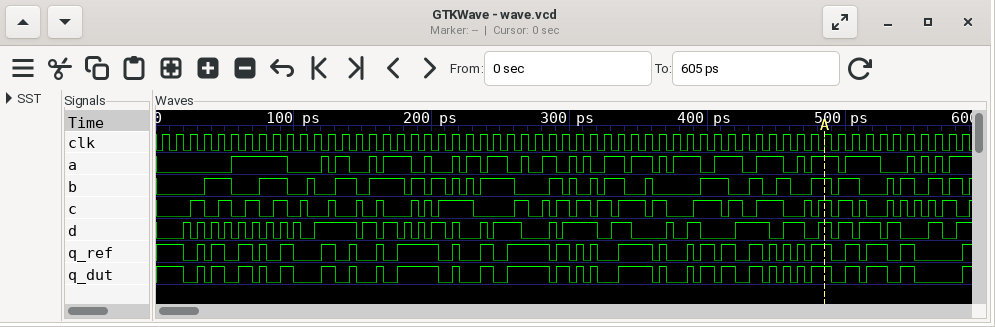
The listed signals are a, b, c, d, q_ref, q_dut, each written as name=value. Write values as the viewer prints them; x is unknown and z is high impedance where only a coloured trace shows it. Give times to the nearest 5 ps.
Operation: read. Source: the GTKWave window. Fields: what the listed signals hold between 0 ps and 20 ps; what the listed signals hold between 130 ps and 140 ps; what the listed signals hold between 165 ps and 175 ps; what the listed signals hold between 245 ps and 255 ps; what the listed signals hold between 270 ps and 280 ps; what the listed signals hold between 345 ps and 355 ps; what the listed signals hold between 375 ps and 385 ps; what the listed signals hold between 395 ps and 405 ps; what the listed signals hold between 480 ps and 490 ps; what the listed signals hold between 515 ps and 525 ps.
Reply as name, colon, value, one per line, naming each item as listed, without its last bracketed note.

what the listed signals hold between 0 ps and 20 ps: a=0, b=0, c=0, d=0, q_ref=1, q_dut=1
what the listed signals hold between 130 ps and 140 ps: a=1, b=1, c=0, d=1, q_ref=0, q_dut=0
what the listed signals hold between 165 ps and 175 ps: a=1, b=1, c=0, d=1, q_ref=0, q_dut=0
what the listed signals hold between 245 ps and 255 ps: a=1, b=1, c=0, d=1, q_ref=0, q_dut=0
what the listed signals hold between 270 ps and 280 ps: a=0, b=0, c=0, d=0, q_ref=1, q_dut=1
what the listed signals hold between 345 ps and 355 ps: a=1, b=0, c=1, d=0, q_ref=1, q_dut=1
what the listed signals hold between 375 ps and 385 ps: a=1, b=0, c=0, d=0, q_ref=0, q_dut=0
what the listed signals hold between 395 ps and 405 ps: a=0, b=1, c=1, d=0, q_ref=1, q_dut=1
what the listed signals hold between 480 ps and 490 ps: a=1, b=1, c=1, d=1, q_ref=1, q_dut=1
what the listed signals hold between 515 ps and 525 ps: a=1, b=0, c=0, d=1, q_ref=1, q_dut=1
